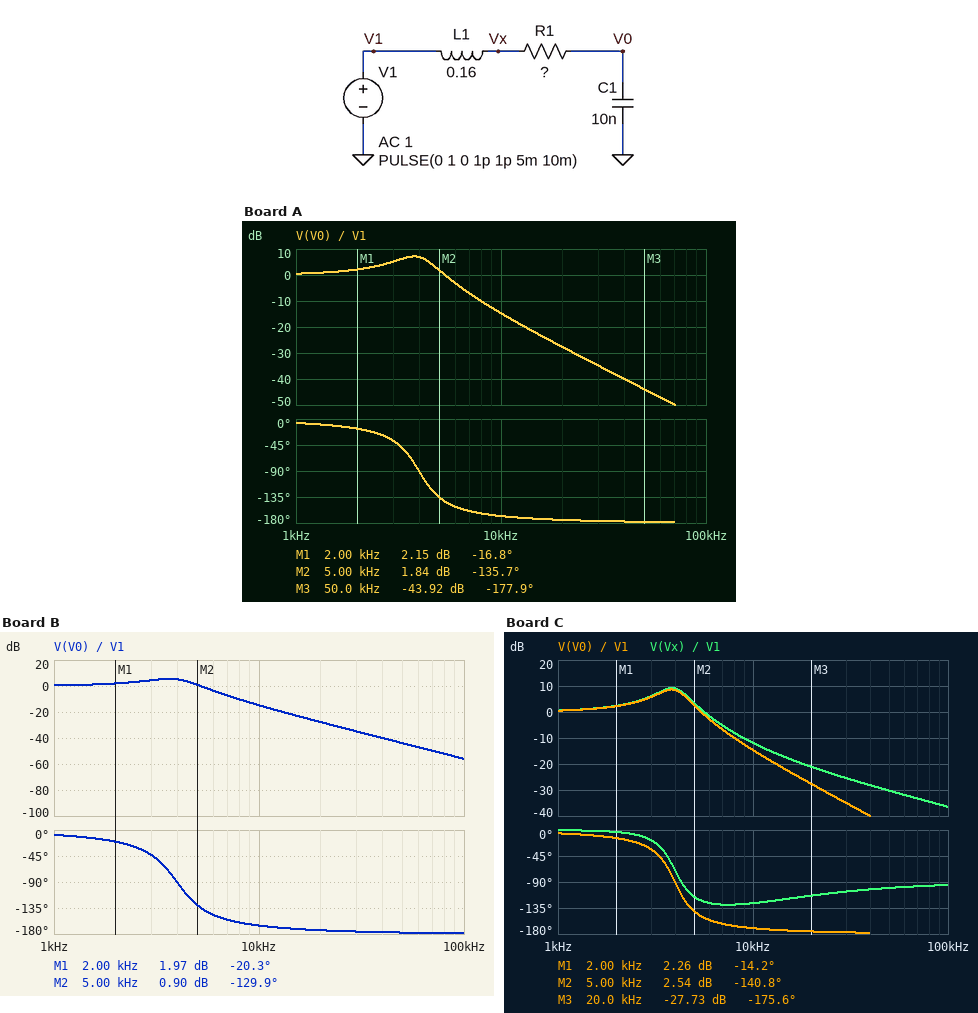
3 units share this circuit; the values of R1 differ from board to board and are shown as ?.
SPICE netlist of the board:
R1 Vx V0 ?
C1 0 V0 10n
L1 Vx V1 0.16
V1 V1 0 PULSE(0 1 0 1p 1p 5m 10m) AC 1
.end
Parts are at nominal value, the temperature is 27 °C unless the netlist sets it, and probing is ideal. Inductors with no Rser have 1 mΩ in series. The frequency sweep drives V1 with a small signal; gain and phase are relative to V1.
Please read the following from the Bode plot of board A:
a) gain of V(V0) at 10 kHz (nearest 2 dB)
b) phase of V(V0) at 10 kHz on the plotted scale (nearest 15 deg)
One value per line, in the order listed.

-14 dB
-165 deg
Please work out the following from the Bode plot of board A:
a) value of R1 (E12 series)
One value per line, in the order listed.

1.8 kΩ
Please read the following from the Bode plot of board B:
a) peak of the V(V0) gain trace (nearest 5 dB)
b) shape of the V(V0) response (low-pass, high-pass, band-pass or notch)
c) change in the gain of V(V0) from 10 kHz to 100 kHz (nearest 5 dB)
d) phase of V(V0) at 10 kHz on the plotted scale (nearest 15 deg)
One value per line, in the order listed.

5 dB
low-pass
-40 dB
-165 deg
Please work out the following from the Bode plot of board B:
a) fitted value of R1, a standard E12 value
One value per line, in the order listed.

2.2 kΩ
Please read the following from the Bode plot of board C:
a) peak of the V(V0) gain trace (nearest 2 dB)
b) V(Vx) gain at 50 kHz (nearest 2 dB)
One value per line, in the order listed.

8 dB
-30 dB
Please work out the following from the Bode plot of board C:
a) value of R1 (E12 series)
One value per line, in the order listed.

1.5 kΩ
